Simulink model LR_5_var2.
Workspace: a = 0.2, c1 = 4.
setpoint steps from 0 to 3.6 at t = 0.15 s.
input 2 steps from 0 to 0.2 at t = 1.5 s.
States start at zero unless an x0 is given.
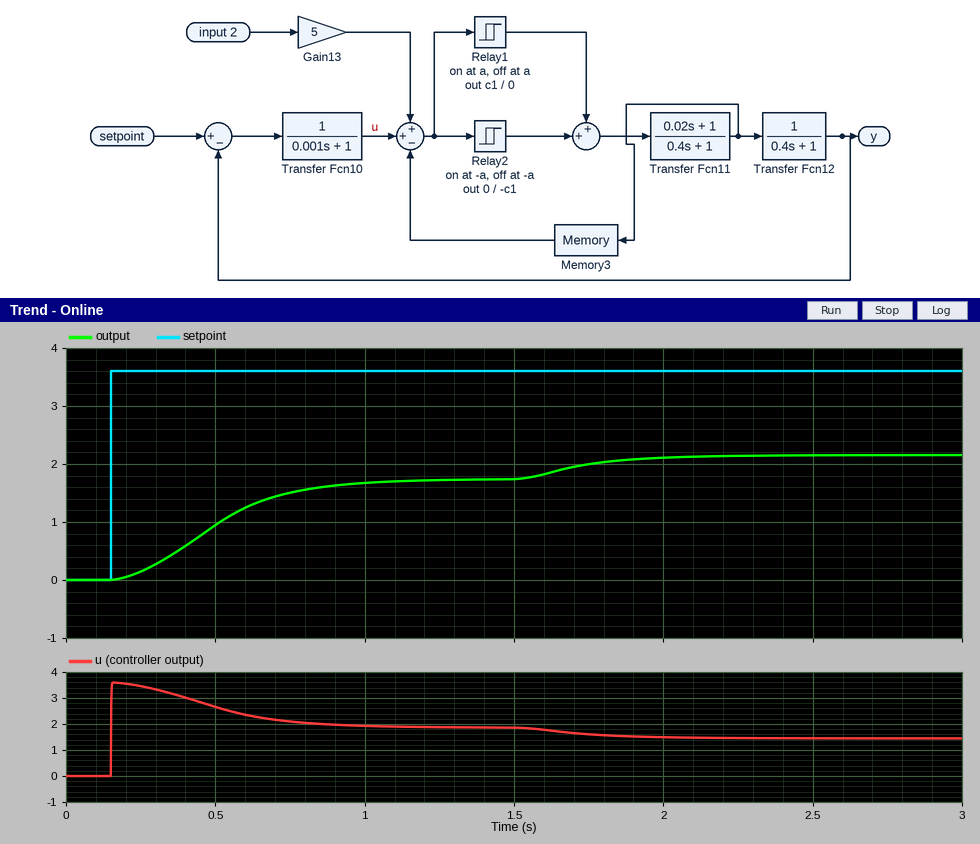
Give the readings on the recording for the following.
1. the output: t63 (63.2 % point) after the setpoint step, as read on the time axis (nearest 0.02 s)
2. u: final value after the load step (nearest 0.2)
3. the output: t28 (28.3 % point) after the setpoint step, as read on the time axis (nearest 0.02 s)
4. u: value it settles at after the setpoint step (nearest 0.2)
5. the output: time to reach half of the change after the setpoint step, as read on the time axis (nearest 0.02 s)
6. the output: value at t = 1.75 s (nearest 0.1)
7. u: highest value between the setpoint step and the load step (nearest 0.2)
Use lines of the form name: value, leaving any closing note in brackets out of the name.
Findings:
the output: t63 (63.2 % point) after the setpoint step, as read on the time axis: 0.54 s
u: final value after the load step: 1.4
the output: t28 (28.3 % point) after the setpoint step, as read on the time axis: 0.38 s
u: value it settles at after the setpoint step: 1.8
the output: time to reach half of the change after the setpoint step, as read on the time axis: 0.48 s
the output: value at t = 1.75 s: 2.0
u: highest value between the setpoint step and the load step: 3.6
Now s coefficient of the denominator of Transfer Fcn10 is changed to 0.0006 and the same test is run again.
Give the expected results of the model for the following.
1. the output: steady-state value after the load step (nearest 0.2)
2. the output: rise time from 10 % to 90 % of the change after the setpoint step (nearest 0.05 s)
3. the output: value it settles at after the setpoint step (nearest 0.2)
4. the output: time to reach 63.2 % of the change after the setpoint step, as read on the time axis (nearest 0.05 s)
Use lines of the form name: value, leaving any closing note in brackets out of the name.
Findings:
the output: steady-state value after the load step: 2.2
the output: rise time from 10 % to 90 % of the change after the setpoint step: 0.55 s
the output: value it settles at after the setpoint step: 1.8
the output: time to reach 63.2 % of the change after the setpoint step, as read on the time axis: 0.55 s
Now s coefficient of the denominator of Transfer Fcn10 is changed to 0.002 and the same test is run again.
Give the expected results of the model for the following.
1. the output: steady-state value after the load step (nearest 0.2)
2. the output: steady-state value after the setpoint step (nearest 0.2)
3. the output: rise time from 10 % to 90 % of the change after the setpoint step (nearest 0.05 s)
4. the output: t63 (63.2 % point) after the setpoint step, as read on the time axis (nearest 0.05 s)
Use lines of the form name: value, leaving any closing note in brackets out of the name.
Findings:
the output: steady-state value after the load step: 2.2
the output: steady-state value after the setpoint step: 1.8
the output: rise time from 10 % to 90 % of the change after the setpoint step: 0.55 s
the output: t63 (63.2 % point) after the setpoint step, as read on the time axis: 0.55 s
